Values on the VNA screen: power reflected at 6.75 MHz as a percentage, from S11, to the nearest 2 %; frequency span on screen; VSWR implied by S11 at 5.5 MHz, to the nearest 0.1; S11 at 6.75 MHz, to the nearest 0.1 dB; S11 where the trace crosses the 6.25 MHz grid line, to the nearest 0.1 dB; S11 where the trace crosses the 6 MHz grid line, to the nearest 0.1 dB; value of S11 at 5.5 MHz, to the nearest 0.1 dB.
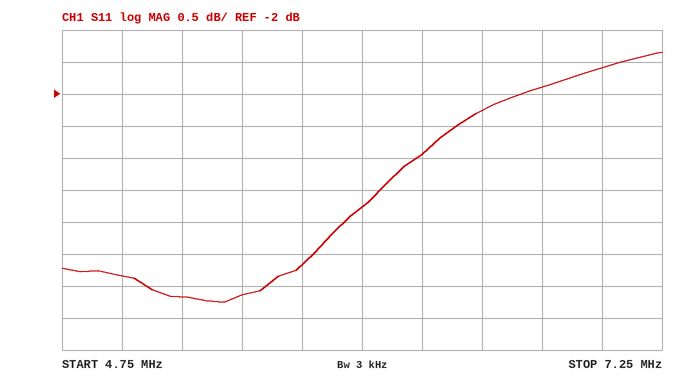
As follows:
64 %
2.5 MHz
3.5
-1.9 dB
-2.9 dB
-3.8 dB
-5.1 dB
